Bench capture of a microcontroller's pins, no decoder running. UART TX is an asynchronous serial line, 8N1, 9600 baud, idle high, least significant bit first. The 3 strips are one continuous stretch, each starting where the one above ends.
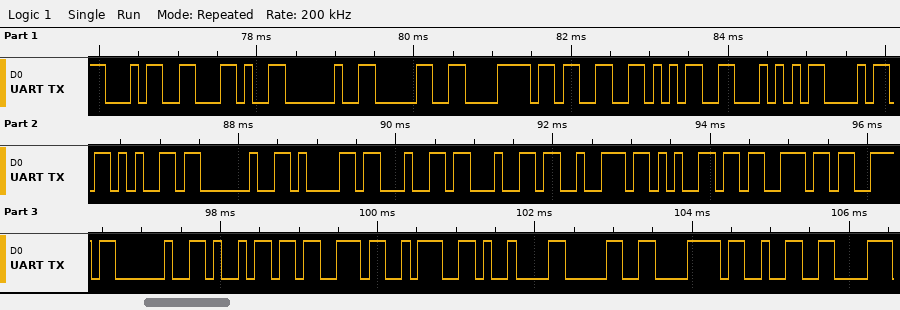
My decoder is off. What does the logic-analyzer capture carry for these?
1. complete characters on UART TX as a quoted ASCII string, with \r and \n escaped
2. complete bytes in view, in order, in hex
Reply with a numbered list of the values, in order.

1. "4, 0x35The address is:\t0x2"
2. 34 2C 20 30 78 33 35 54 68 65 20 61 64 64 72 65 73 73 20 69 73 3A 09 30 78 32
